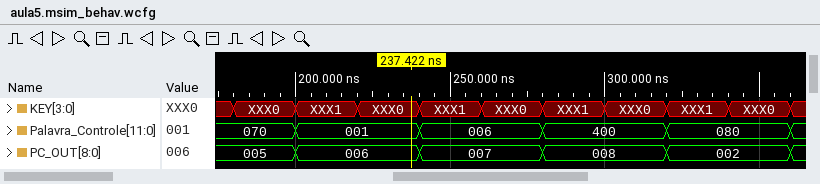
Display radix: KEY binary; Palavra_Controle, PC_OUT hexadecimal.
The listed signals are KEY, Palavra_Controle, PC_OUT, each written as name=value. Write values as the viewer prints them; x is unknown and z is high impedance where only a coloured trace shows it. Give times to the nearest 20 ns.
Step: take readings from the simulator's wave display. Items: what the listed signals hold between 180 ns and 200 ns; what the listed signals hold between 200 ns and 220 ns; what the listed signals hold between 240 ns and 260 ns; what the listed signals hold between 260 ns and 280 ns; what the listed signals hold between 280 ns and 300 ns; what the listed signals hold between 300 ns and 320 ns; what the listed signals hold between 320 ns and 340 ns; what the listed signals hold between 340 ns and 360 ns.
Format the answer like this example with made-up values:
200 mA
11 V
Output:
KEY=XXX0, Palavra_Controle=070, PC_OUT=005
KEY=XXX1, Palavra_Controle=001, PC_OUT=006
KEY=XXX1, Palavra_Controle=006, PC_OUT=007
KEY=XXX0, Palavra_Controle=006, PC_OUT=007
KEY=XXX1, Palavra_Controle=400, PC_OUT=008
KEY=XXX0, Palavra_Controle=400, PC_OUT=008
KEY=XXX1, Palavra_Controle=080, PC_OUT=002
KEY=XXX0, Palavra_Controle=080, PC_OUT=002
